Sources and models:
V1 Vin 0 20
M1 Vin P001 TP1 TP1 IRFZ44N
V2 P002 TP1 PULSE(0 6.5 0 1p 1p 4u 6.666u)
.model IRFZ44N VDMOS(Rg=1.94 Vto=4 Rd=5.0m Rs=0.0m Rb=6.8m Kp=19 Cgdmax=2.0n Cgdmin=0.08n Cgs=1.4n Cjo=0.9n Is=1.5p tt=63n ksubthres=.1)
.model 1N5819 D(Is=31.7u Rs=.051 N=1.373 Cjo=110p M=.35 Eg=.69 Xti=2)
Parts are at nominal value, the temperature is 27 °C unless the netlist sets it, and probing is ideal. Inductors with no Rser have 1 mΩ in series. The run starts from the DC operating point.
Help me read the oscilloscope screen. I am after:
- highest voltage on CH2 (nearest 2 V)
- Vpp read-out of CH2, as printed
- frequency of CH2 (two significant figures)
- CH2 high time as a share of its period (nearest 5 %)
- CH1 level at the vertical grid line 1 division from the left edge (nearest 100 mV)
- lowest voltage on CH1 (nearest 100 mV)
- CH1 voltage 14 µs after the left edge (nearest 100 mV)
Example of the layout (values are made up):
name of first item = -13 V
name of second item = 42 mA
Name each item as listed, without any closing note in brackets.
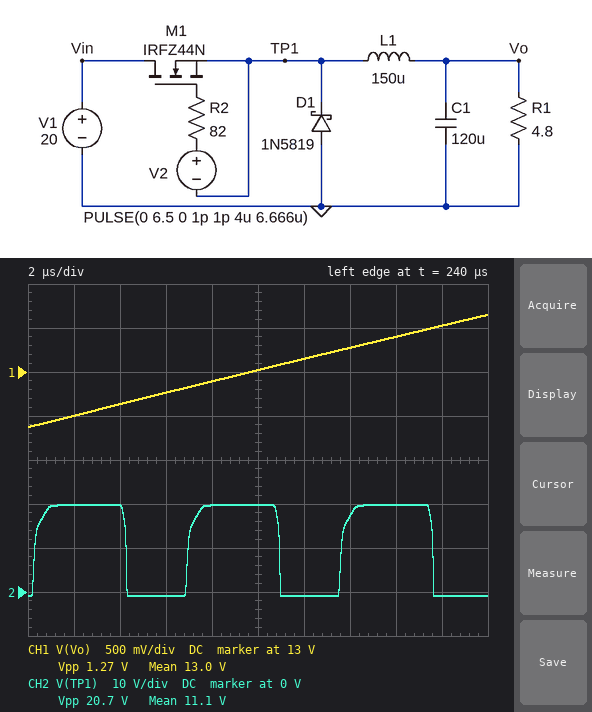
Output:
highest voltage on CH2 = 20 V
Vpp read-out of CH2, as printed = 20.7 V
frequency of CH2 = 150 kHz
CH2 high time as a share of its period = 60 %
CH1 level at the vertical grid line 1 division from the left edge = 12.5 V
lowest voltage on CH1 = 12.4 V
CH1 voltage 14 µs after the left edge = 13.3 V
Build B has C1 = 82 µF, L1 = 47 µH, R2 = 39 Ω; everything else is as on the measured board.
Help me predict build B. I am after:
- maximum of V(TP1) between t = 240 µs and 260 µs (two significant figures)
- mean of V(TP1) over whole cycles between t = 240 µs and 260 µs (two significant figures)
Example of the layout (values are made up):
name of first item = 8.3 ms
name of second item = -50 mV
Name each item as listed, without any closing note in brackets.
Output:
maximum of V(TP1) between t = 240 µs and 260 µs = 21 V
mean of V(TP1) over whole cycles between t = 240 µs and 260 µs = 18 V
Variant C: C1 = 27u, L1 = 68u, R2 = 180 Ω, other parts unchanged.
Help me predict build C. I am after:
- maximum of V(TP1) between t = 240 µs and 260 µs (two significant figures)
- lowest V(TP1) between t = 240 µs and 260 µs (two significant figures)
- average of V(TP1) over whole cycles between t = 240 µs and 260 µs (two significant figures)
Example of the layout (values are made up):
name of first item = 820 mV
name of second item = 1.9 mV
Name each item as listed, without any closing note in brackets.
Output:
maximum of V(TP1) between t = 240 µs and 260 µs = 20 V
lowest V(TP1) between t = 240 µs and 260 µs = -470 mV
average of V(TP1) over whole cycles between t = 240 µs and 260 µs = 12 V
